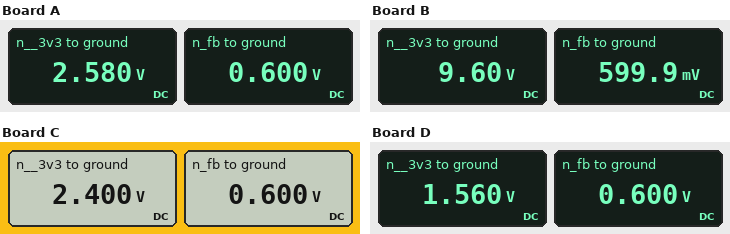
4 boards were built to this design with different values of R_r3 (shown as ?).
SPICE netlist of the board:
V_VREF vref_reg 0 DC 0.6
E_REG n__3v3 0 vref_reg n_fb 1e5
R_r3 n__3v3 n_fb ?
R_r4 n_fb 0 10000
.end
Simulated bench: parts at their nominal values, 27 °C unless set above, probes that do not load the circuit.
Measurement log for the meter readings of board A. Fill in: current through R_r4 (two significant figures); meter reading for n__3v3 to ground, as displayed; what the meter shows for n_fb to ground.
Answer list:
60 µA
2.580 V
0.600 V
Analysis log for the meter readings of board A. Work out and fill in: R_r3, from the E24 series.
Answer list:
33 kΩ
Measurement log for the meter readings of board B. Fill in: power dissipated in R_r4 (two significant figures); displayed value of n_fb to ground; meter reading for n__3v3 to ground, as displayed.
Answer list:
36 µW
599.9 mV
9.60 V
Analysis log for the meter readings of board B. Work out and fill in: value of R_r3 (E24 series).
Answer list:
150 kΩ
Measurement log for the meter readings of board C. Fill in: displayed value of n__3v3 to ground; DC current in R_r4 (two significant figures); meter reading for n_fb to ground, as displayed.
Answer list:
2.400 V
60 µA
0.600 V
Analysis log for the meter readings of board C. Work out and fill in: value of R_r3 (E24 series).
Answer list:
30 kΩ
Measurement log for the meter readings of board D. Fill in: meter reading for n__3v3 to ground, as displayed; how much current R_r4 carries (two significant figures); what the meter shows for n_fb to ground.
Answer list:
1.560 V
60 µA
0.600 V
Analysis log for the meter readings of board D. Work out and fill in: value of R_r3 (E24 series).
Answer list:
16 kΩ
